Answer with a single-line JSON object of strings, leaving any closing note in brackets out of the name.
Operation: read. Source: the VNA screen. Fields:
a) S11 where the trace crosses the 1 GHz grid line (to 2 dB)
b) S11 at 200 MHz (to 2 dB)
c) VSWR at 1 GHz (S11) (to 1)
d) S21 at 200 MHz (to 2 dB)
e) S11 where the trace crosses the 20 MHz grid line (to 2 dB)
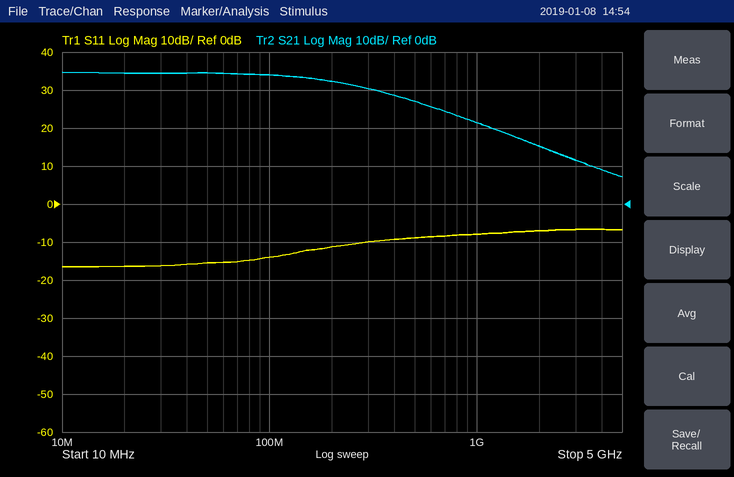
{"S11 where the trace crosses the 1 GHz grid line": "-8 dB", "S11 at 200 MHz": "-12 dB", "VSWR at 1 GHz (S11)": "2", "S21 at 200 MHz": "32 dB", "S11 where the trace crosses the 20 MHz grid line": "-16 dB"}
